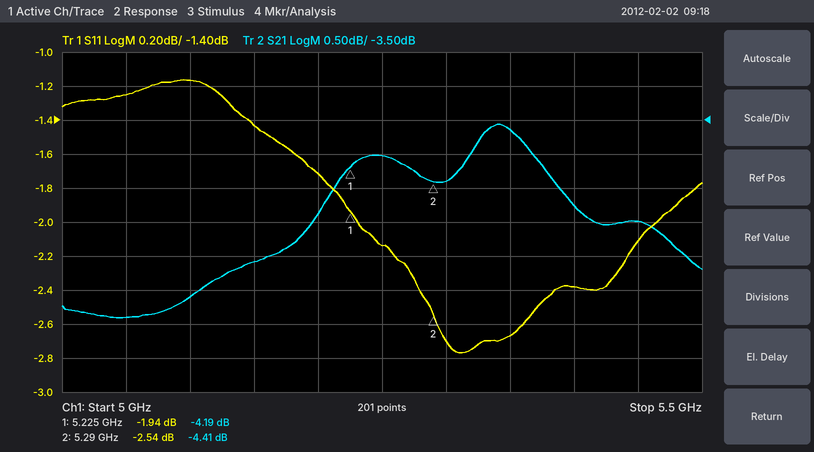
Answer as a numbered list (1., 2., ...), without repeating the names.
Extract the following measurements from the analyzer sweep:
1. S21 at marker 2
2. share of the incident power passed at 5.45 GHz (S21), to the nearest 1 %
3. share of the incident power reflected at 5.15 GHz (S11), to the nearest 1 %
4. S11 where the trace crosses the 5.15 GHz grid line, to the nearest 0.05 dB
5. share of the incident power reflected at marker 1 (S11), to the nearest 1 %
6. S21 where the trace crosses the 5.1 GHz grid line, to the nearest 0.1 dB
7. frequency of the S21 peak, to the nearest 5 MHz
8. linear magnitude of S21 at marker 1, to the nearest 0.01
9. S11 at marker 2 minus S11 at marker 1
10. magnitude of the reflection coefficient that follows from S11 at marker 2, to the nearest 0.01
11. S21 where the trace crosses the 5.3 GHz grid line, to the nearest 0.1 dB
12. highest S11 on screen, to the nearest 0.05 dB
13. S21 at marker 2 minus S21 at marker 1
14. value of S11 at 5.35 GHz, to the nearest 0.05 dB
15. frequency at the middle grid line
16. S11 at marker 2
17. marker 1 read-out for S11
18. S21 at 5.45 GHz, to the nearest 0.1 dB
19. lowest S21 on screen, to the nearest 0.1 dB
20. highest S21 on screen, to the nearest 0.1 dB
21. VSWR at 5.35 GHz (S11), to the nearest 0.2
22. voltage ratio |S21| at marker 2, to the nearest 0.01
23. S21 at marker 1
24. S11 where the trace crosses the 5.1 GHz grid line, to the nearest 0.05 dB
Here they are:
1. -4.41 dB
2. 32 %
3. 72 %
4. -1.45 dB
5. 64 %
6. -6.1 dB
7. 5.340 GHz
8. 0.62
9. -0.60 dB
10. 0.75
11. -4.4 dB
12. -1.15 dB
13. -0.22 dB
14. -2.65 dB
15. 5.25 GHz
16. -2.54 dB
17. -1.94 dB
18. -5.0 dB
19. -6.4 dB
20. -3.6 dB
21. 6.6
22. 0.60
23. -4.19 dB
24. -1.15 dB
